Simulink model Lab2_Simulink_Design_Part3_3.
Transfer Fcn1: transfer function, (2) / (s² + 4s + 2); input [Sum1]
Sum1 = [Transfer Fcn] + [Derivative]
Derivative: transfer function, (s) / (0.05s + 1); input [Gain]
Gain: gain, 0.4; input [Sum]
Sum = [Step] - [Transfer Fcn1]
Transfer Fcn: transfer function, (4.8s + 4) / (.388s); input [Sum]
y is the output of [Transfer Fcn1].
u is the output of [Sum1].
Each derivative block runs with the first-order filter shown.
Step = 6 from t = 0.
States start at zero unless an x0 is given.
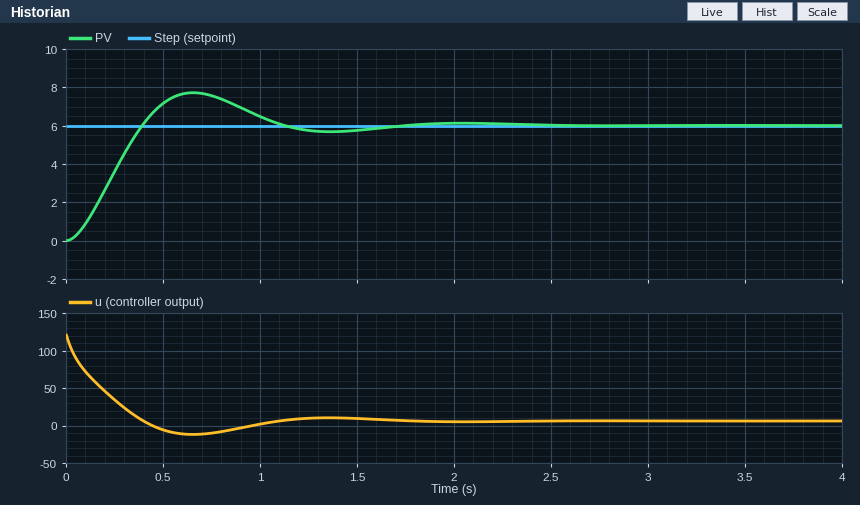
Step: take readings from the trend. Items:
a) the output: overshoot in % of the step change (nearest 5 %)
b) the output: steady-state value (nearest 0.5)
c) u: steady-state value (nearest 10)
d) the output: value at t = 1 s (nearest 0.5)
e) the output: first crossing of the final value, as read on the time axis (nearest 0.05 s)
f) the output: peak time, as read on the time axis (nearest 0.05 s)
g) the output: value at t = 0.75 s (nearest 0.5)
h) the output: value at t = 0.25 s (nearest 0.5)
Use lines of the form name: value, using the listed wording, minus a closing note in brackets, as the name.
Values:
the output: overshoot in % of the step change: 30 %
the output: steady-state value: 6.0
u: steady-state value: 10
the output: value at t = 1 s: 6.5
the output: first crossing of the final value, as read on the time axis: 0.40 s
the output: peak time, as read on the time axis: 0.65 s
the output: value at t = 0.75 s: 7.5
the output: value at t = 0.25 s: 3.5
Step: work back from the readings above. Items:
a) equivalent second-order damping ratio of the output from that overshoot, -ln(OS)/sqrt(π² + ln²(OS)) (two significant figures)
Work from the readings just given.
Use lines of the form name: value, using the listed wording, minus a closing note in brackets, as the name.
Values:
equivalent second-order damping ratio of the output from that overshoot, -ln(OS)/sqrt(π² + ln²(OS)): 0.36
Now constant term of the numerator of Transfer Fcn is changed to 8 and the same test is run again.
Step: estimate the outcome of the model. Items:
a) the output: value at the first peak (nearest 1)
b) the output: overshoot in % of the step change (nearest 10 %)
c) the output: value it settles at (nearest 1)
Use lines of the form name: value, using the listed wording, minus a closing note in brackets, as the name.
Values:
the output: value at the first peak: 9
the output: overshoot in % of the step change: 40 %
the output: value it settles at: 6
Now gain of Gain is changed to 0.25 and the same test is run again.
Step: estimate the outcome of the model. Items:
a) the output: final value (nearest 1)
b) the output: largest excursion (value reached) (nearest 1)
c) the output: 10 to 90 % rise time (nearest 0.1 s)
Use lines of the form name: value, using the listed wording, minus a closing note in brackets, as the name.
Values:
the output: final value: 6
the output: largest excursion (value reached): 8
the output: 10 to 90 % rise time: 0.3 s
